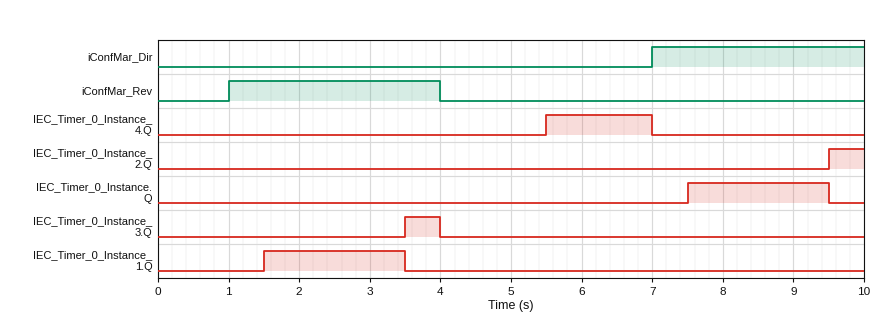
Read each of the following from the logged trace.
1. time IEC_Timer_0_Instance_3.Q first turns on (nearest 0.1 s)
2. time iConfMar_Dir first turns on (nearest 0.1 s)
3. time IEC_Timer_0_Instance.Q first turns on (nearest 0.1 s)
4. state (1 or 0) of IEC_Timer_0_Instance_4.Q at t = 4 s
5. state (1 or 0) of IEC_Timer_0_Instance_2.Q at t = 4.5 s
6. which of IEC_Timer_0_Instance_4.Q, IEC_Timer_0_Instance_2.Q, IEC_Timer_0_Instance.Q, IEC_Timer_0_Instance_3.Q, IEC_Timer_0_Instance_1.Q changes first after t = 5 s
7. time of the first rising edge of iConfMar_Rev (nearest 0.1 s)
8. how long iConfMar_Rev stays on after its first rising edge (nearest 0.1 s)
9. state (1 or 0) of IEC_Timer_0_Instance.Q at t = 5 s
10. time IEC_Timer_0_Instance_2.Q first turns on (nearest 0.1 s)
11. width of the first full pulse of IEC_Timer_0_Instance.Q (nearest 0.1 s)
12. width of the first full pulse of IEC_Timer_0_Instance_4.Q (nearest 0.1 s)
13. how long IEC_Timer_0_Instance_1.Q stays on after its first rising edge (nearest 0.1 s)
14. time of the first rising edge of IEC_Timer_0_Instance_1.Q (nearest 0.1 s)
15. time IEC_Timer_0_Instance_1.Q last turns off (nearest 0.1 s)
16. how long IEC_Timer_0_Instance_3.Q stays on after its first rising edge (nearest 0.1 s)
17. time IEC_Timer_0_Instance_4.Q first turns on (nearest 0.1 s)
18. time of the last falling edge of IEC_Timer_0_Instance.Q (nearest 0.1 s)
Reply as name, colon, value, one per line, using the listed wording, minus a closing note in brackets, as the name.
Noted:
time IEC_Timer_0_Instance_3.Q first turns on: 3.5 s
time iConfMar_Dir first turns on: 7.0 s
time IEC_Timer_0_Instance.Q first turns on: 7.5 s
state (1 or 0) of IEC_Timer_0_Instance_4.Q at t = 4 s: 0
state (1 or 0) of IEC_Timer_0_Instance_2.Q at t = 4.5 s: 0
which of IEC_Timer_0_Instance_4.Q, IEC_Timer_0_Instance_2.Q, IEC_Timer_0_Instance.Q, IEC_Timer_0_Instance_3.Q, IEC_Timer_0_Instance_1.Q changes first after t = 5 s: IEC_Timer_0_Instance_4.Q
time of the first rising edge of iConfMar_Rev: 1.0 s
how long iConfMar_Rev stays on after its first rising edge: 3.0 s
state (1 or 0) of IEC_Timer_0_Instance.Q at t = 5 s: 0
time IEC_Timer_0_Instance_2.Q first turns on: 9.5 s
width of the first full pulse of IEC_Timer_0_Instance.Q: 2.0 s
width of the first full pulse of IEC_Timer_0_Instance_4.Q: 1.5 s
how long IEC_Timer_0_Instance_1.Q stays on after its first rising edge: 2.0 s
time of the first rising edge of IEC_Timer_0_Instance_1.Q: 1.5 s
time IEC_Timer_0_Instance_1.Q last turns off: 3.5 s
how long IEC_Timer_0_Instance_3.Q stays on after its first rising edge: 0.5 s
time IEC_Timer_0_Instance_4.Q first turns on: 5.5 s
time of the last falling edge of IEC_Timer_0_Instance.Q: 9.5 s
